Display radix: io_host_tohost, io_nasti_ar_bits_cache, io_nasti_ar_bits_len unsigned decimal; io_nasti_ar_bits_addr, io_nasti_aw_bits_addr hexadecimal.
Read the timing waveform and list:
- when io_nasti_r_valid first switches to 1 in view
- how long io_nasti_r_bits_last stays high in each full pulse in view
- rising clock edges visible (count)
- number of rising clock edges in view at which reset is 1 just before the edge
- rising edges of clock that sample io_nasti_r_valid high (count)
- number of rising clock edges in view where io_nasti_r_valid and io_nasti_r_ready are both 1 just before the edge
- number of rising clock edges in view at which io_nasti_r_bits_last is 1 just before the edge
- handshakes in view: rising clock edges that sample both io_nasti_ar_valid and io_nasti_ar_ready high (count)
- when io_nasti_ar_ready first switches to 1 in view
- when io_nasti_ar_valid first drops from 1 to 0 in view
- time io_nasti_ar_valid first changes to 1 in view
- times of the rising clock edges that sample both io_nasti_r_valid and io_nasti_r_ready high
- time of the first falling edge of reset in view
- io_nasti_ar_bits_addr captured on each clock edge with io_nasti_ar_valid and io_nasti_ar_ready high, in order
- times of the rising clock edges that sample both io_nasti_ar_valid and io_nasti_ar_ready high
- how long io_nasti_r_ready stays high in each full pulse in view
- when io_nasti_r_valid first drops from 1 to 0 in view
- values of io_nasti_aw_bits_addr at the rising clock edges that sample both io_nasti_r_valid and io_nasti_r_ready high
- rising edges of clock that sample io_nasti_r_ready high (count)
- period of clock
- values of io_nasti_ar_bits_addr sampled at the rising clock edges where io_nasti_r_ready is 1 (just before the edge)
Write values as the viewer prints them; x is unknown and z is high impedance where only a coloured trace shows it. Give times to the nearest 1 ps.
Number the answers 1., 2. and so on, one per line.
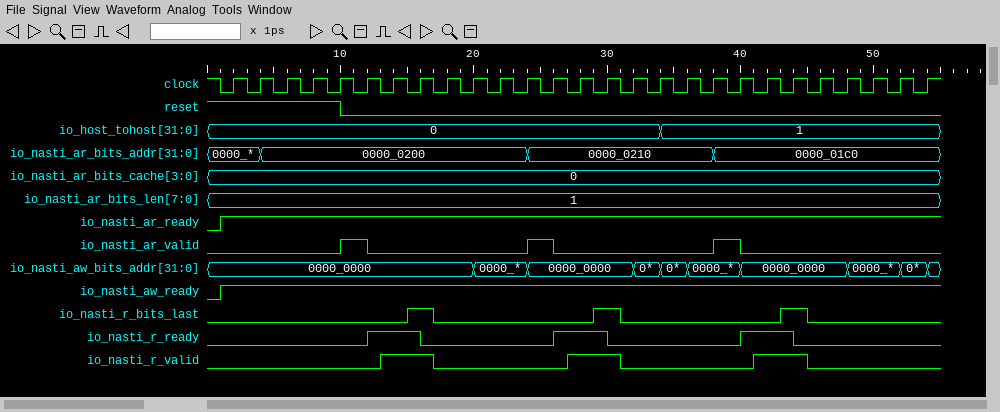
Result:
1. 13 ps
2. 2 ps, 2 ps, 2 ps
3. 27
4. 5
5. 6
6. 6
7. 3
8. 3
9. 1 ps
10. 12 ps
11. 10 ps
12. 14 ps, 16 ps, 28 ps, 30 ps, 42 ps, 44 ps
13. 10 ps
14. 0000_0200, 0000_0210, 0000_01c0
15. 12 ps, 26 ps, 40 ps
16. 4 ps, 4 ps, 4 ps
17. 17 ps
18. 0000_0000, 0000_0000, 0000_0000, 0000_0000, 0000_0000, 0000_0000
19. 6
20. 2 ps
21. 0000_0200, 0000_0200, 0000_0210, 0000_0210, 0000_01c0, 0000_01c0
